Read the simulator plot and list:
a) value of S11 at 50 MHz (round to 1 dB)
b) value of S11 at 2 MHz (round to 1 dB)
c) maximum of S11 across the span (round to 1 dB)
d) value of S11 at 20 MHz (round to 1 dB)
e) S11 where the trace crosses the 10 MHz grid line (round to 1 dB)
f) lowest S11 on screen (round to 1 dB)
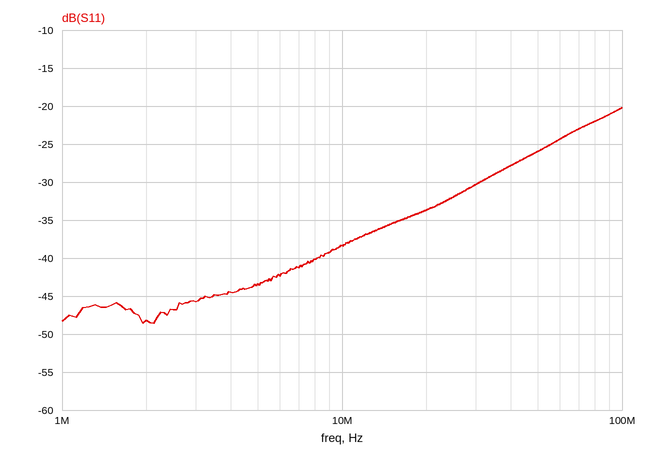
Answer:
-26 dB
-48 dB
-20 dB
-34 dB
-38 dB
-49 dB
